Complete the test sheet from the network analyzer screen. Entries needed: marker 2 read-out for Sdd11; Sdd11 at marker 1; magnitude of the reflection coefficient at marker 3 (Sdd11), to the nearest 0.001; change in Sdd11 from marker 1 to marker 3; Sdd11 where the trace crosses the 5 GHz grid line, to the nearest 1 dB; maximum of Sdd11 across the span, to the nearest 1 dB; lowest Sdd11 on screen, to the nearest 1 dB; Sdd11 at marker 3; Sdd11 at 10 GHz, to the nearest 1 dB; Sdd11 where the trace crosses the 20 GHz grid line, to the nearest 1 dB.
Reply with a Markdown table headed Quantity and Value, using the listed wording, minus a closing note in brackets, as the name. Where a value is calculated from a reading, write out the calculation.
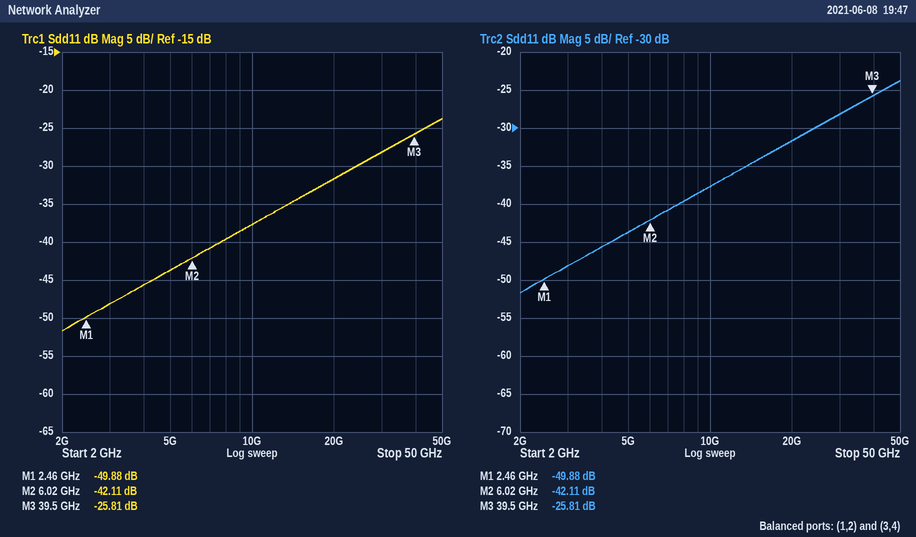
| Quantity | Value |
|---|---|
| marker 2 read-out for Sdd11 | -42.11 dB |
| Sdd11 at marker 1 | -49.88 dB |
| magnitude of the reflection coefficient at marker 3 (Sdd11), to the nearest 0.001 | 10^(-25.81/20) ≈ 0.051 |
| change in Sdd11 from marker 1 to marker 3 | -25.81 − (-49.88) = 24.07 dB |
| Sdd11 where the trace crosses the 5 GHz grid line, to the nearest 1 dB | -44 dB |
| maximum of Sdd11 across the span, to the nearest 1 dB | -24 dB |
| lowest Sdd11 on screen, to the nearest 1 dB | -52 dB |
| Sdd11 at marker 3 | -25.81 dB |
| Sdd11 at 10 GHz, to the nearest 1 dB | -38 dB |
| Sdd11 where the trace crosses the 20 GHz grid line, to the nearest 1 dB | -32 dB |
